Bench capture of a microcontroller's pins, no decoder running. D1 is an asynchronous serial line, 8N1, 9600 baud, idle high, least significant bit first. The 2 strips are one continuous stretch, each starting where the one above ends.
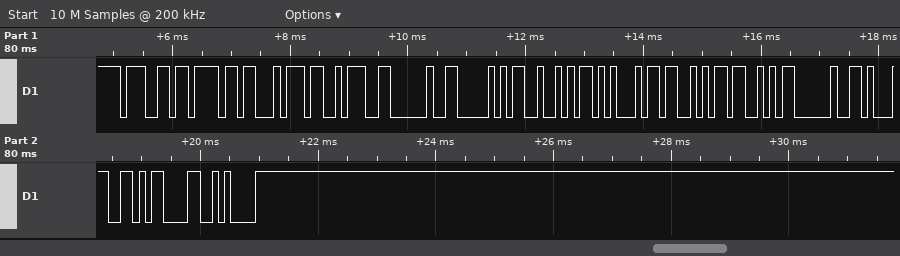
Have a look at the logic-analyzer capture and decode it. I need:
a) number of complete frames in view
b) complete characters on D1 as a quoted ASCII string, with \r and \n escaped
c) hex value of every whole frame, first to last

14
"got: PRESS 1\r\n"
67 6F 74 3A 20 50 52 45 53 53 20 31 0D 0A
